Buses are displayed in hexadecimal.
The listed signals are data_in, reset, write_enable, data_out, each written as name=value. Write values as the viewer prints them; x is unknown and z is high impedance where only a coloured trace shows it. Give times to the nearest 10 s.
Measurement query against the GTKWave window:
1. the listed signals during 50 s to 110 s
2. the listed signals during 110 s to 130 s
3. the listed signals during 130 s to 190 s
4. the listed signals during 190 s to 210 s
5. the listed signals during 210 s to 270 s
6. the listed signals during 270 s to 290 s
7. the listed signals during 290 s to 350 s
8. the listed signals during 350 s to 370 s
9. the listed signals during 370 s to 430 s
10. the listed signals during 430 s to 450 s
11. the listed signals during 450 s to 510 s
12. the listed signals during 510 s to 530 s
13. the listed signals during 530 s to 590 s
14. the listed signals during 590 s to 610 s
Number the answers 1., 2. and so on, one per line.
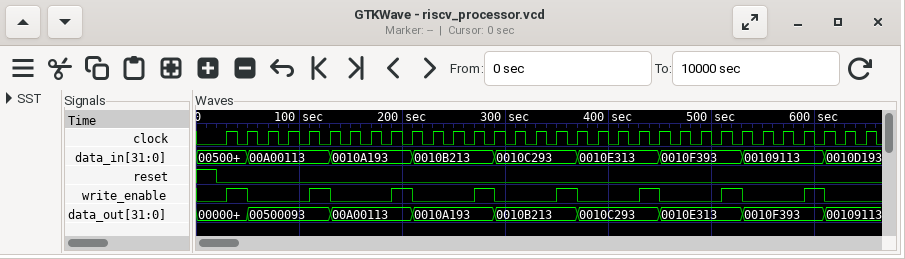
1. data_in=00A00113, reset=0, write_enable=0, data_out=00500093
2. data_in=00A00113, reset=0, write_enable=1, data_out=00500093
3. data_in=0010A193, reset=0, write_enable=0, data_out=00A00113
4. data_in=0010A193, reset=0, write_enable=1, data_out=00A00113
5. data_in=0010B213, reset=0, write_enable=0, data_out=0010A193
6. data_in=0010B213, reset=0, write_enable=1, data_out=0010A193
7. data_in=0010C293, reset=0, write_enable=0, data_out=0010B213
8. data_in=0010C293, reset=0, write_enable=1, data_out=0010B213
9. data_in=0010E313, reset=0, write_enable=0, data_out=0010C293
10. data_in=0010E313, reset=0, write_enable=1, data_out=0010C293
11. data_in=0010F393, reset=0, write_enable=0, data_out=0010E313
12. data_in=0010F393, reset=0, write_enable=1, data_out=0010E313
13. data_in=00109113, reset=0, write_enable=0, data_out=0010F393
14. data_in=00109113, reset=0, write_enable=1, data_out=0010F393
